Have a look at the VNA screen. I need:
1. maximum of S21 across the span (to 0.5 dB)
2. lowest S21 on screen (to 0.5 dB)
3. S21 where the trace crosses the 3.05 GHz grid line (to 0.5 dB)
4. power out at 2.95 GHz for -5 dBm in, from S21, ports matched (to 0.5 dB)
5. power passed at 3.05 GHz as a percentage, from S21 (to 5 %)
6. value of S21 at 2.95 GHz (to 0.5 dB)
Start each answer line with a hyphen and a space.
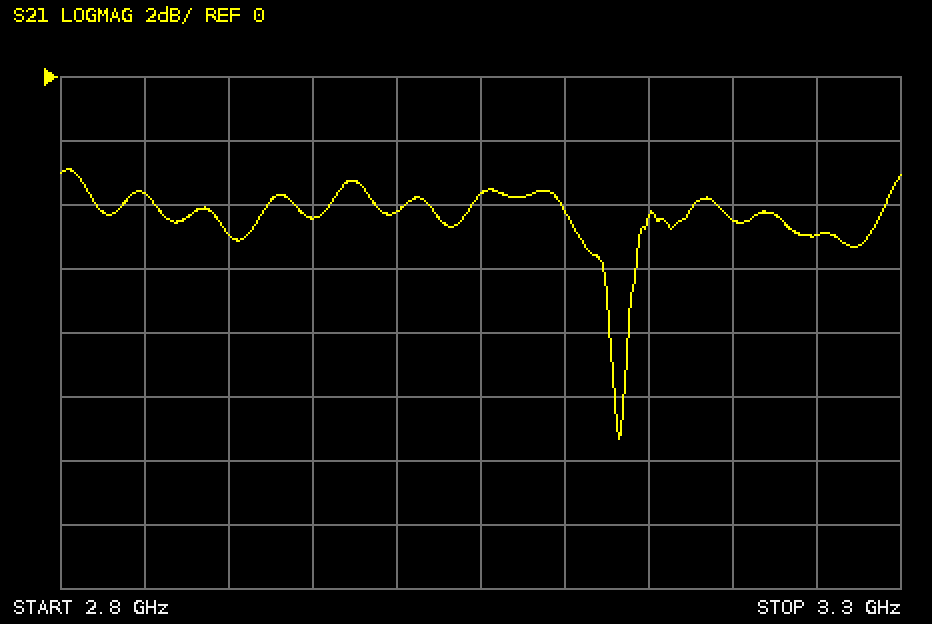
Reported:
- -3.0 dB
- -11.5 dB
- -3.5 dB
- -9.5 dBm
- 45 %
- -4.5 dB
